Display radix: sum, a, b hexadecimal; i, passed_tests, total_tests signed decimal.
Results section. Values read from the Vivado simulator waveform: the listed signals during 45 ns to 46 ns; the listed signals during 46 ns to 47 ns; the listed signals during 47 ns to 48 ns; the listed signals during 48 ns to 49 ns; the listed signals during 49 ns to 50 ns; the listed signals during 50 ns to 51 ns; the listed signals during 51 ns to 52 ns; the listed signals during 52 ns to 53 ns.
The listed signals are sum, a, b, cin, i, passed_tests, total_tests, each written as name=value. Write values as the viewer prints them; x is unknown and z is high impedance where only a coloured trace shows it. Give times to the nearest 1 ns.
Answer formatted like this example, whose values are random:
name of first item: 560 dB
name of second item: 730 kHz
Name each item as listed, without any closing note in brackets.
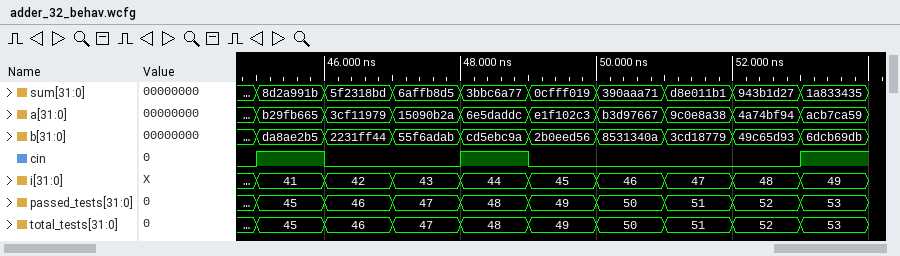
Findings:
the listed signals during 45 ns to 46 ns: sum=8d2a991b, a=b29fb665, b=da8ae2b5, cin=1, i=41, passed_tests=45, total_tests=45
the listed signals during 46 ns to 47 ns: sum=5f2318bd, a=3cf11979, b=2231ff44, cin=0, i=42, passed_tests=46, total_tests=46
the listed signals during 47 ns to 48 ns: sum=6affb8d5, a=15090b2a, b=55f6adab, cin=0, i=43, passed_tests=47, total_tests=47
the listed signals during 48 ns to 49 ns: sum=3bbc6a77, a=6e5daddc, b=cd5ebc9a, cin=1, i=44, passed_tests=48, total_tests=48
the listed signals during 49 ns to 50 ns: sum=0cfff019, a=e1f102c3, b=2b0eed56, cin=0, i=45, passed_tests=49, total_tests=49
the listed signals during 50 ns to 51 ns: sum=390aaa71, a=b3d97667, b=8531340a, cin=0, i=46, passed_tests=50, total_tests=50
the listed signals during 51 ns to 52 ns: sum=d8e011b1, a=9c0e8a38, b=3cd18779, cin=0, i=47, passed_tests=51, total_tests=51
the listed signals during 52 ns to 53 ns: sum=943b1d27, a=4a74bf94, b=49c65d93, cin=0, i=48, passed_tests=52, total_tests=52
